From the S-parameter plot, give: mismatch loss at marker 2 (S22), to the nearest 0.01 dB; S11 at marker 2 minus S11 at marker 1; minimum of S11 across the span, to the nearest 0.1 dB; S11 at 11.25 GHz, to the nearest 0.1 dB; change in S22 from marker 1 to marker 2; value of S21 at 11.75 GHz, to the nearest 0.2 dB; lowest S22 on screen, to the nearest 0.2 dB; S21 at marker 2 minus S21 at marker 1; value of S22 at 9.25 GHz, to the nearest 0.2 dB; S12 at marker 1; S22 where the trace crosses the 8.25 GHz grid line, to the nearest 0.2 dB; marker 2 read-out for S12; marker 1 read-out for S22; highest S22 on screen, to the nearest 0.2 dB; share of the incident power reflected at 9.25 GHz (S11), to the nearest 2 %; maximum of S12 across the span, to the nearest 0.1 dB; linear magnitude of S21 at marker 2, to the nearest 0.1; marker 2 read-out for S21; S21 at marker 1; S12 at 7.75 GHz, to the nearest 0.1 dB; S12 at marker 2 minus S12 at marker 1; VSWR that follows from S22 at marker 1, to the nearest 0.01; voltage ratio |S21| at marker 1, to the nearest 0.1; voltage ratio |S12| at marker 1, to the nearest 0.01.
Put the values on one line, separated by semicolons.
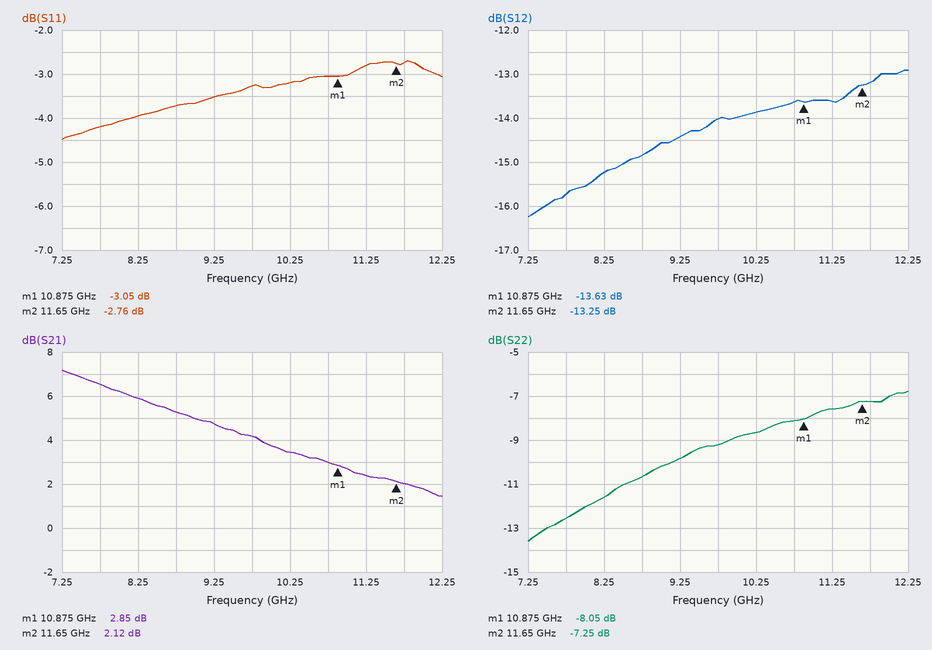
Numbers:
0.91 dB; 0.29 dB; -4.5 dB; -2.8 dB; 0.80 dB; 2.0 dB; -13.6 dB; -0.73 dB; -9.8 dB; -13.63 dB; -11.6 dB; -13.25 dB; -8.05 dB; -6.8 dB; 44 %; -12.9 dB; 1.3; 2.12 dB; 2.85 dB; -15.7 dB; 0.38 dB; 2.31; 1.4; 0.21
